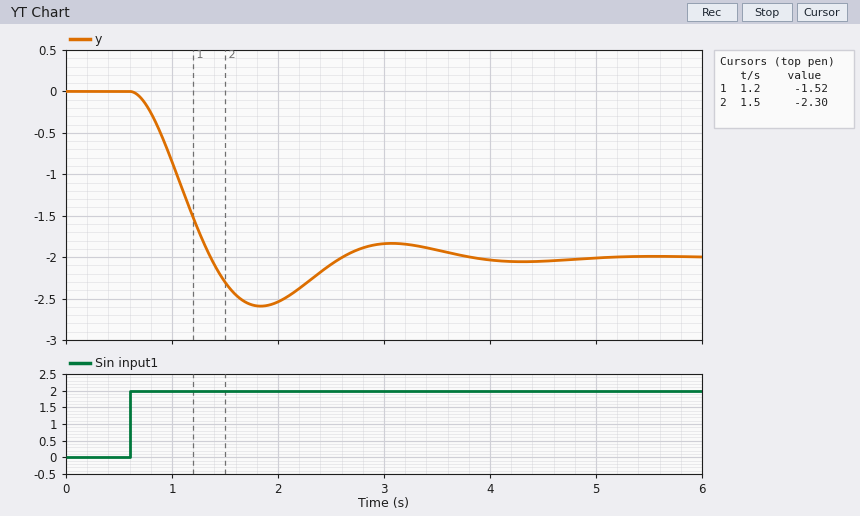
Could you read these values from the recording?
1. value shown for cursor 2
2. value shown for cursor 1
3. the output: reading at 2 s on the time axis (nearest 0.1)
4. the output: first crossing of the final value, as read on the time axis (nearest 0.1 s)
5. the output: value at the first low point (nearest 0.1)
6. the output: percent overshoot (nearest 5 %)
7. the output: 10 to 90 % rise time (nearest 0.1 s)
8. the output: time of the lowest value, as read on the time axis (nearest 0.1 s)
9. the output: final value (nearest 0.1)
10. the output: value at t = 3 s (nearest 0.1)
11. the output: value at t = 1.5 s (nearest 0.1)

-2.30
-1.52
-2.5
1.4 s
-2.6
30 %
0.5 s
1.8 s
-2.0
-1.8
-2.3
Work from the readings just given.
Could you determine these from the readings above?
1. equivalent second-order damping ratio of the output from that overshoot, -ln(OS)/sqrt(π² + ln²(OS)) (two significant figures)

0.36
